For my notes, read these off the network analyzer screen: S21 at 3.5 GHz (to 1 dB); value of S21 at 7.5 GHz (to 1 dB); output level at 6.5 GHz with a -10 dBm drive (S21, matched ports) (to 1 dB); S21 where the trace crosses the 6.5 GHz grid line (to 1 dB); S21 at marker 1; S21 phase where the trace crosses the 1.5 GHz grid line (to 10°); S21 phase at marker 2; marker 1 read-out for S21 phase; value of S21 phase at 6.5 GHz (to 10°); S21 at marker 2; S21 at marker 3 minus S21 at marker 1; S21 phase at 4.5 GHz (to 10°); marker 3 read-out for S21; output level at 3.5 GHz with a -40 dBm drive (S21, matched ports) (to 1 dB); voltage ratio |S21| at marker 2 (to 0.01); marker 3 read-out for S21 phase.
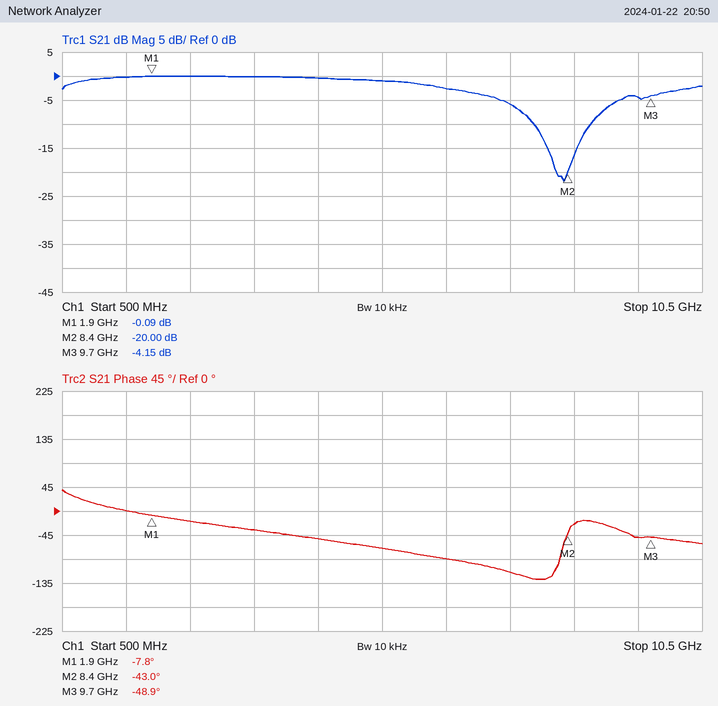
0 dB
-6 dB
-13 dBm
-3 dB
-0.09 dB
0°
-43.0°
-7.8°
-90°
-20.00 dB
-4.06 dB
-50°
-4.15 dB
-40 dBm
0.10
-48.9°
